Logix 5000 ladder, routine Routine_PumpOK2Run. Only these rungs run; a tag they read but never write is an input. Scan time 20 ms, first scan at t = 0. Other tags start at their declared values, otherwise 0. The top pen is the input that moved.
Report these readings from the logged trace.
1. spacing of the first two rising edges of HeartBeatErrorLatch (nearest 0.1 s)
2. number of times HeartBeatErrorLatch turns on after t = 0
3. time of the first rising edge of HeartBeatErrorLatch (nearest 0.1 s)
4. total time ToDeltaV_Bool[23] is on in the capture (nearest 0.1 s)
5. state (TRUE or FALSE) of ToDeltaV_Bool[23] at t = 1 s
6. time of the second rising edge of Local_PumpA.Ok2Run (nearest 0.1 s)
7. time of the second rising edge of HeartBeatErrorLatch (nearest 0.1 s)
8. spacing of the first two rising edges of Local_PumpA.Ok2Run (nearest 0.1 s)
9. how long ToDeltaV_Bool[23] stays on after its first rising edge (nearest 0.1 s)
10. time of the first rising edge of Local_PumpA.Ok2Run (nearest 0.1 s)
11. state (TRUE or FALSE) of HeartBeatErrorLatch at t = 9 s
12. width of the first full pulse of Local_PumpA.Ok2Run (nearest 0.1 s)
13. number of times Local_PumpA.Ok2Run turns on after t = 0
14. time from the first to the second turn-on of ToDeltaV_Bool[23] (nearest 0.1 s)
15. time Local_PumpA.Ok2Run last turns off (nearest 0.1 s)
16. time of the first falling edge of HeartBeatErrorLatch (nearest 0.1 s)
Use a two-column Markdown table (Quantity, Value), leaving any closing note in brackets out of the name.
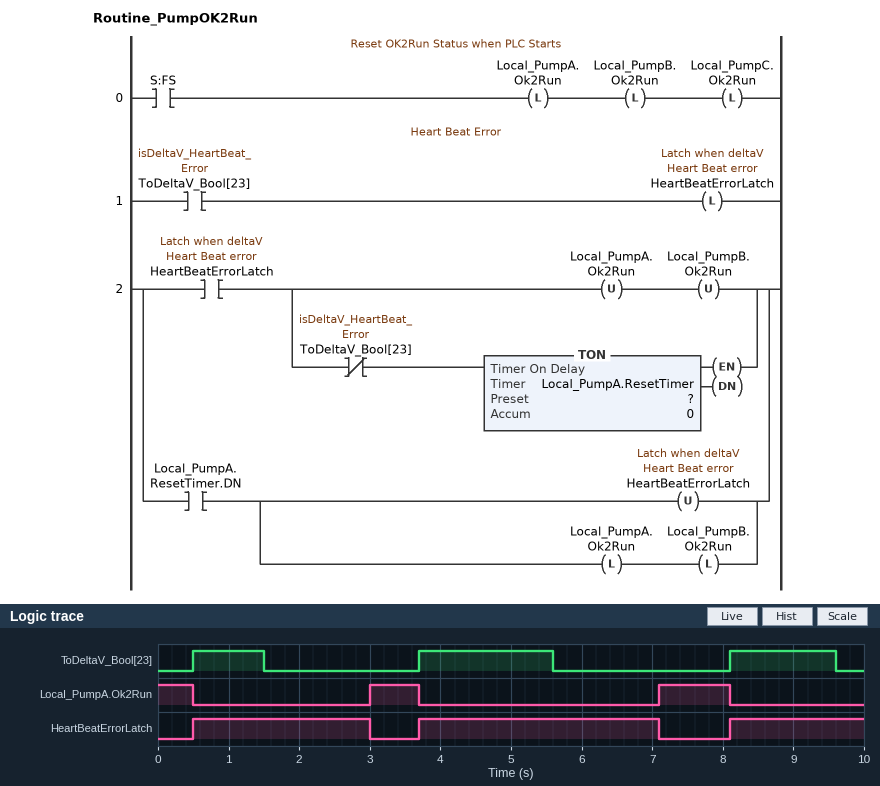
| Quantity | Value |
|---|---|
| spacing of the first two rising edges of HeartBeatErrorLatch | 3.2 s |
| number of times HeartBeatErrorLatch turns on after t = 0 | 3 |
| time of the first rising edge of HeartBeatErrorLatch | 0.5 s |
| total time ToDeltaV_Bool[23] is on in the capture | 4.4 s |
| state (TRUE or FALSE) of ToDeltaV_Bool[23] at t = 1 s | TRUE |
| time of the second rising edge of Local_PumpA.Ok2Run | 7.1 s |
| time of the second rising edge of HeartBeatErrorLatch | 3.7 s |
| spacing of the first two rising edges of Local_PumpA.Ok2Run | 4.1 s |
| how long ToDeltaV_Bool[23] stays on after its first rising edge | 1.0 s |
| time of the first rising edge of Local_PumpA.Ok2Run | 3.0 s |
| state (TRUE or FALSE) of HeartBeatErrorLatch at t = 9 s | TRUE |
| width of the first full pulse of Local_PumpA.Ok2Run | 0.7 s |
| number of times Local_PumpA.Ok2Run turns on after t = 0 | 2 |
| time from the first to the second turn-on of ToDeltaV_Bool[23] | 3.2 s |
| time Local_PumpA.Ok2Run last turns off | 8.1 s |
| time of the first falling edge of HeartBeatErrorLatch | 3.0 s |
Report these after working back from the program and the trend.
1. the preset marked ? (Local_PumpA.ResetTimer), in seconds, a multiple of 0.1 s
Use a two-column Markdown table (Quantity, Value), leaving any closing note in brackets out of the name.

| Quantity | Value |
|---|---|
| the preset marked ? (Local_PumpA.ResetTimer), in seconds, a multiple of 0.1 s | 1.5 s |
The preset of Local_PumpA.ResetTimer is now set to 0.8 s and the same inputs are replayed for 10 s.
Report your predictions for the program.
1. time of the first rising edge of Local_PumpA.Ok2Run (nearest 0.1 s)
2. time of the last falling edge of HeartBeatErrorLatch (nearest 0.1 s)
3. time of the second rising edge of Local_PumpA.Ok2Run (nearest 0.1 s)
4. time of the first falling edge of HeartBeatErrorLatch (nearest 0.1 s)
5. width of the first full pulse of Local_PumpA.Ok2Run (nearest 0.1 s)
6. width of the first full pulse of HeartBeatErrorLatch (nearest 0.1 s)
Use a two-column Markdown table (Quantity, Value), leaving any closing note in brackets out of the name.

| Quantity | Value |
|---|---|
| time of the first rising edge of Local_PumpA.Ok2Run | 2.3 s |
| time of the last falling edge of HeartBeatErrorLatch | 6.4 s |
| time of the second rising edge of Local_PumpA.Ok2Run | 6.4 s |
| time of the first falling edge of HeartBeatErrorLatch | 2.3 s |
| width of the first full pulse of Local_PumpA.Ok2Run | 1.4 s |
| width of the first full pulse of HeartBeatErrorLatch | 1.8 s |
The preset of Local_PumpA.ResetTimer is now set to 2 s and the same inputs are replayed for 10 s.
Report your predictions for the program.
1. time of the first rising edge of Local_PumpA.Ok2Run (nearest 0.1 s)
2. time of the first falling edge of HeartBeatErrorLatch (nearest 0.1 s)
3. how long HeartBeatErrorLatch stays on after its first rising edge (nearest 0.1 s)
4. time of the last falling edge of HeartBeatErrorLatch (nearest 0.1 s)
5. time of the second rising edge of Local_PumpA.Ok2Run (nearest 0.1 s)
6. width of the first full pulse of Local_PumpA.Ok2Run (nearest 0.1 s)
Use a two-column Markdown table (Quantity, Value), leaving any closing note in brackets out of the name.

| Quantity | Value |
|---|---|
| time of the first rising edge of Local_PumpA.Ok2Run | 3.5 s |
| time of the first falling edge of HeartBeatErrorLatch | 3.5 s |
| how long HeartBeatErrorLatch stays on after its first rising edge | 3.0 s |
| time of the last falling edge of HeartBeatErrorLatch | 7.6 s |
| time of the second rising edge of Local_PumpA.Ok2Run | 7.6 s |
| width of the first full pulse of Local_PumpA.Ok2Run | 0.2 s |
